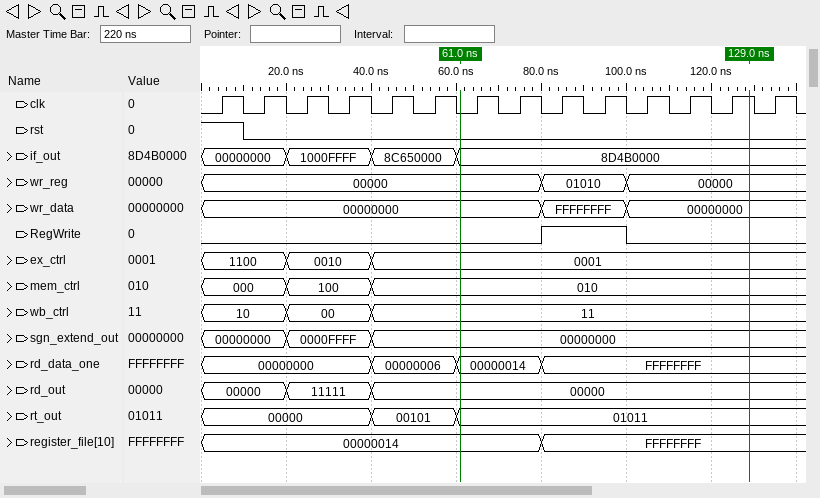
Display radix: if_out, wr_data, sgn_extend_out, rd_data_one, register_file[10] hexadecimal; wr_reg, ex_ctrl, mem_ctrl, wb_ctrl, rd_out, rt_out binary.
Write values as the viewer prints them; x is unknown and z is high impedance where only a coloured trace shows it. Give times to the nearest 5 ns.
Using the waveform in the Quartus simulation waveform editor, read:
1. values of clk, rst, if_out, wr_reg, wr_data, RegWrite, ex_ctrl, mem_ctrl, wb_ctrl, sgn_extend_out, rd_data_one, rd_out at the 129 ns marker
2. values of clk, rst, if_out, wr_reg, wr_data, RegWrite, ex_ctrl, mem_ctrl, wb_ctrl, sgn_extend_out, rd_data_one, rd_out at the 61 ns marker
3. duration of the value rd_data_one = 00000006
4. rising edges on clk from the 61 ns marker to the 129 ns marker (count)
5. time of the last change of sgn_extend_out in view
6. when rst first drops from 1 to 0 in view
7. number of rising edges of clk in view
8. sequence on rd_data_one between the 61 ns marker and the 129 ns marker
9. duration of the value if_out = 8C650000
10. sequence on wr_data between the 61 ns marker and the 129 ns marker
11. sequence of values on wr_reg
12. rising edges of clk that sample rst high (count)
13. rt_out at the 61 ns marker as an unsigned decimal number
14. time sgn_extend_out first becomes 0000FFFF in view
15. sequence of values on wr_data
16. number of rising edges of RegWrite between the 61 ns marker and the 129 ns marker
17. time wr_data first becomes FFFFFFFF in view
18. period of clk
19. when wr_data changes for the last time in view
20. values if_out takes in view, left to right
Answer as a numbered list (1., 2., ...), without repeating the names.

1. clk=1, rst=0, if_out=8D4B0000, wr_reg=00000, wr_data=00000000, RegWrite=0, ex_ctrl=0001, mem_ctrl=010, wb_ctrl=11, sgn_extend_out=00000000, rd_data_one=FFFFFFFF, rd_out=00000
2. clk=0, rst=0, if_out=8D4B0000, wr_reg=00000, wr_data=00000000, RegWrite=0, ex_ctrl=0001, mem_ctrl=010, wb_ctrl=11, sgn_extend_out=00000000, rd_data_one=00000014, rd_out=00000
3. 20 ns
4. 7
5. 40 ns
6. 10 ns
7. 14
8. 00000014, FFFFFFFF
9. 20 ns
10. 00000000, FFFFFFFF, 00000000
11. 00000, 01010, 00000
12. 1
13. 11
14. 20 ns
15. 00000000, FFFFFFFF, 00000000
16. 1
17. 80 ns
18. 10 ns
19. 100 ns
20. 00000000, 1000FFFF, 8C650000, 8D4B0000
